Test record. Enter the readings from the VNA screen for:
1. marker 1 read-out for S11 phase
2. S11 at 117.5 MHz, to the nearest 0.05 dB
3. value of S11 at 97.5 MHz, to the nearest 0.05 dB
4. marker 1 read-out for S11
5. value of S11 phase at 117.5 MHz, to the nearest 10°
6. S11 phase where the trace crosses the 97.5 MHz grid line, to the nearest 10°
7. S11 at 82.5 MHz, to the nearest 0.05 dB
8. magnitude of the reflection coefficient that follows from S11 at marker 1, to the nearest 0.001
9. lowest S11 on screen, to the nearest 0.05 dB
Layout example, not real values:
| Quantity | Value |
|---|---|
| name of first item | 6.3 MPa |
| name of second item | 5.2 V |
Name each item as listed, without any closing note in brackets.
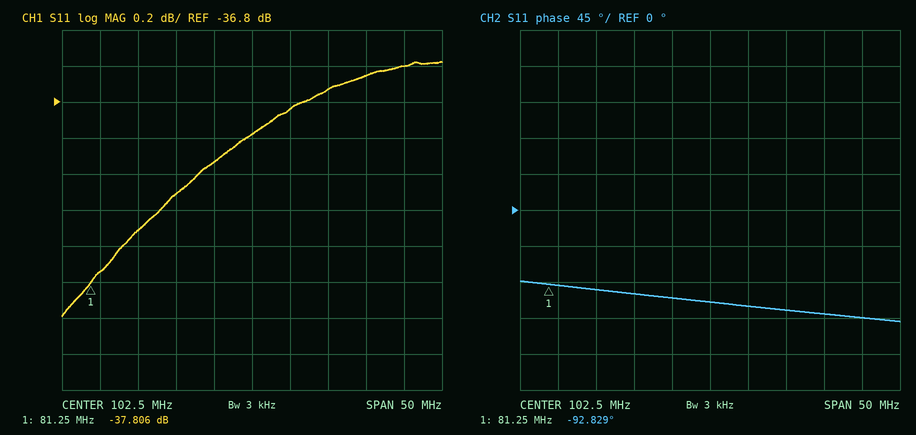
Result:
| Quantity | Value |
|---|---|
| marker 1 read-out for S11 phase | -92.829° |
| S11 at 117.5 MHz, to the nearest 0.05 dB | -36.65 dB |
| value of S11 at 97.5 MHz, to the nearest 0.05 dB | -37.15 dB |
| marker 1 read-out for S11 | -37.806 dB |
| value of S11 phase at 117.5 MHz, to the nearest 10° | -130° |
| S11 phase where the trace crosses the 97.5 MHz grid line, to the nearest 10° | -110° |
| S11 at 82.5 MHz, to the nearest 0.05 dB | -37.75 dB |
| magnitude of the reflection coefficient that follows from S11 at marker 1, to the nearest 0.001 | 0.013 |
| lowest S11 on screen, to the nearest 0.05 dB | -38.00 dB |
